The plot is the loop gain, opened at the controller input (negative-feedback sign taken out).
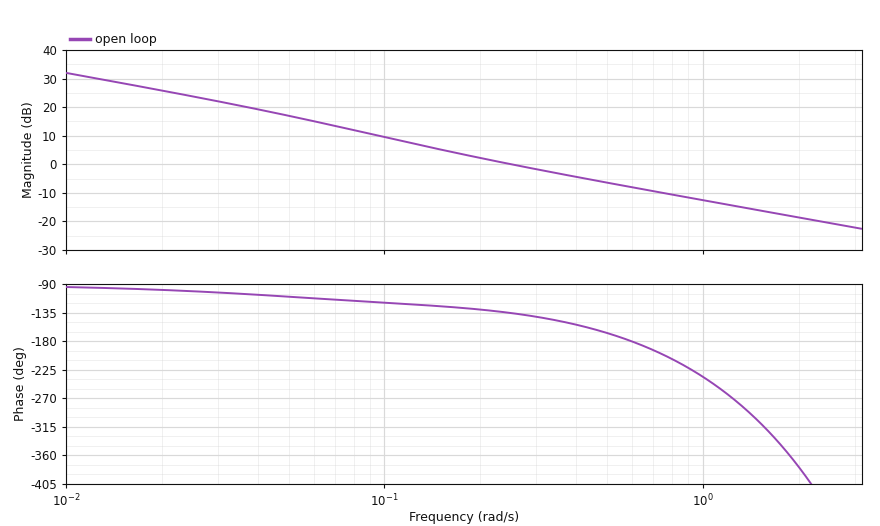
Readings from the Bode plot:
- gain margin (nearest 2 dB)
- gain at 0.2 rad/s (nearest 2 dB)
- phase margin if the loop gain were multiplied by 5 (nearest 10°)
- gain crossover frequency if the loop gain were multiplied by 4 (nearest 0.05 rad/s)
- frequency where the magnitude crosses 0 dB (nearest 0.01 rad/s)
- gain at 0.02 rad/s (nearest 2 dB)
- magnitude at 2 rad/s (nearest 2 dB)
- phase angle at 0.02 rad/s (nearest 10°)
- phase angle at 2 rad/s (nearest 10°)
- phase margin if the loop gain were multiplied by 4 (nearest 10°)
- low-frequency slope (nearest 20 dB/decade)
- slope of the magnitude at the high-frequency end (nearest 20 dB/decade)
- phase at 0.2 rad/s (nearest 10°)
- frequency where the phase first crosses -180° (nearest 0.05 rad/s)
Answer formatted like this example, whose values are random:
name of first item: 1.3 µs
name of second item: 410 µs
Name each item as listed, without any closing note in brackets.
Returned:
gain margin: 8 dB
gain at 0.2 rad/s: 2 dB
phase margin if the loop gain were multiplied by 5: -80°
gain crossover frequency if the loop gain were multiplied by 4: 0.95 rad/s
frequency where the magnitude crosses 0 dB: 0.25 rad/s
gain at 0.02 rad/s: 26 dB
magnitude at 2 rad/s: -18 dB
phase angle at 0.02 rad/s: -100°
phase angle at 2 rad/s: -380°
phase margin if the loop gain were multiplied by 4: -50°
low-frequency slope: -20 dB/decade
slope of the magnitude at the high-frequency end: -20 dB/decade
phase at 0.2 rad/s: -130°
frequency where the phase first crosses -180°: 0.60 rad/s
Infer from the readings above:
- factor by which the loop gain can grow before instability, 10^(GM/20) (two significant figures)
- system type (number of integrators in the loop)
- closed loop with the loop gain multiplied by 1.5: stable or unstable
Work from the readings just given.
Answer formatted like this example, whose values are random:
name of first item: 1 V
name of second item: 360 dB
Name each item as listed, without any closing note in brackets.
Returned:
factor by which the loop gain can grow before instability, 10^(GM/20): 2.5
system type: 1
closed loop with the loop gain multiplied by 1.5: stable or unstable: stable
